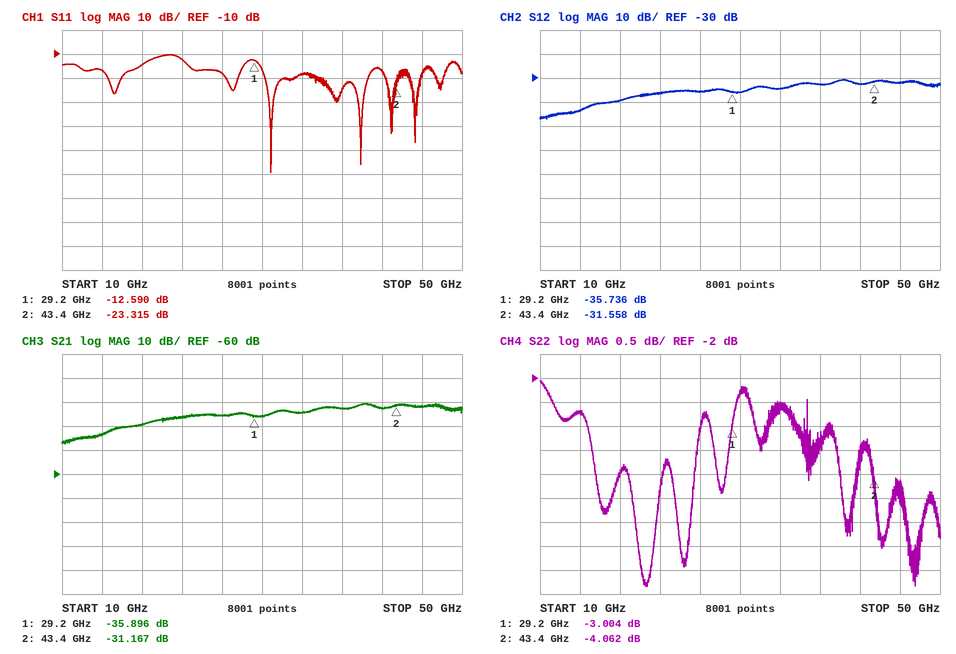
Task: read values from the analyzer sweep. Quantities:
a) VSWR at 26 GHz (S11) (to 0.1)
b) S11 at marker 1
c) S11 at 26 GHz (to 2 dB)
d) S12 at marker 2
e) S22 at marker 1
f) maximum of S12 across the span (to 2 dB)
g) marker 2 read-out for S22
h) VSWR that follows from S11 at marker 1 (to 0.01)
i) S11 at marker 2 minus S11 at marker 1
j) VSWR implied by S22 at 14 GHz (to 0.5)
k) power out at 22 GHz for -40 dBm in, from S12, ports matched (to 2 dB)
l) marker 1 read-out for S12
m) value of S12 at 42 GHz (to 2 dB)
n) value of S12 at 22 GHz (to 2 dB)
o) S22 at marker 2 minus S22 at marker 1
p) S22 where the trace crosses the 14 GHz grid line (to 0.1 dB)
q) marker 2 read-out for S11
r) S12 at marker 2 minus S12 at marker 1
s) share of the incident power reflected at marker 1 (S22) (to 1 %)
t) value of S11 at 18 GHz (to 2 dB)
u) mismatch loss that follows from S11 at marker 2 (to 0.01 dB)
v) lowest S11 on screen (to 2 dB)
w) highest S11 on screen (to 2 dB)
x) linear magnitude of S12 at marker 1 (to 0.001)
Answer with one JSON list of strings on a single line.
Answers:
["1.3", "-12.590 dB", "-18 dB", "-31.558 dB", "-3.004 dB", "-30 dB", "-4.062 dB", "1.61", "-10.725 dB", "6.5", "-76 dBm", "-35.736 dB", "-32 dB", "-36 dB", "-1.058 dB", "-2.7 dB", "-23.315 dB", "4.178 dB", "50 %", "-14 dB", "0.02 dB", "-60 dB", "-10 dB", "0.016"]
